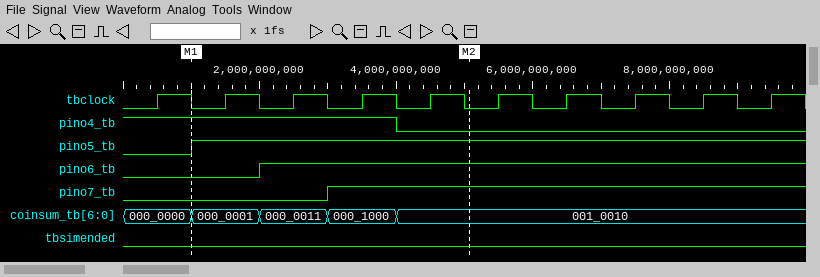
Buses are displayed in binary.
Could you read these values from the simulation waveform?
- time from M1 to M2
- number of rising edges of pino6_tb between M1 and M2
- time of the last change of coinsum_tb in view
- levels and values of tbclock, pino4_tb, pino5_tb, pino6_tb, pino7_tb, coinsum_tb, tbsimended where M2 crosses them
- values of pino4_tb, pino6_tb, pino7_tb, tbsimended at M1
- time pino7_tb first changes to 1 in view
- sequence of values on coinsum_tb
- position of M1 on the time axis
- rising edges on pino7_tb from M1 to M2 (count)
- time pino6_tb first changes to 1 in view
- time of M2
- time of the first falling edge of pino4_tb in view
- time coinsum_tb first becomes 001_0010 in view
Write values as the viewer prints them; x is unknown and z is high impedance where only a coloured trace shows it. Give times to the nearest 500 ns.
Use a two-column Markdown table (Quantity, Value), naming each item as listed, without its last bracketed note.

| Quantity | Value |
|---|---|
| time from M1 to M2 | 4000 ns |
| number of rising edges of pino6_tb between M1 and M2 | 1 |
| time of the last change of coinsum_tb in view | 4000 ns |
| levels and values of tbclock, pino4_tb, pino5_tb, pino6_tb, pino7_tb, coinsum_tb, tbsimended where M2 crosses them | tbclock=0, pino4_tb=0, pino5_tb=1, pino6_tb=1, pino7_tb=1, coinsum_tb=001_0010, tbsimended=0 |
| values of pino4_tb, pino6_tb, pino7_tb, tbsimended at M1 | pino4_tb=1, pino6_tb=0, pino7_tb=0, tbsimended=0 |
| time pino7_tb first changes to 1 in view | 3000 ns |
| sequence of values on coinsum_tb | 000_0000, 000_0001, 000_0011, 000_1000, 001_0010 |
| position of M1 on the time axis | 1000 ns |
| rising edges on pino7_tb from M1 to M2 | 1 |
| time pino6_tb first changes to 1 in view | 2000 ns |
| time of M2 | 5000 ns |
| time of the first falling edge of pino4_tb in view | 4000 ns |
| time coinsum_tb first becomes 001_0010 in view | 4000 ns |
